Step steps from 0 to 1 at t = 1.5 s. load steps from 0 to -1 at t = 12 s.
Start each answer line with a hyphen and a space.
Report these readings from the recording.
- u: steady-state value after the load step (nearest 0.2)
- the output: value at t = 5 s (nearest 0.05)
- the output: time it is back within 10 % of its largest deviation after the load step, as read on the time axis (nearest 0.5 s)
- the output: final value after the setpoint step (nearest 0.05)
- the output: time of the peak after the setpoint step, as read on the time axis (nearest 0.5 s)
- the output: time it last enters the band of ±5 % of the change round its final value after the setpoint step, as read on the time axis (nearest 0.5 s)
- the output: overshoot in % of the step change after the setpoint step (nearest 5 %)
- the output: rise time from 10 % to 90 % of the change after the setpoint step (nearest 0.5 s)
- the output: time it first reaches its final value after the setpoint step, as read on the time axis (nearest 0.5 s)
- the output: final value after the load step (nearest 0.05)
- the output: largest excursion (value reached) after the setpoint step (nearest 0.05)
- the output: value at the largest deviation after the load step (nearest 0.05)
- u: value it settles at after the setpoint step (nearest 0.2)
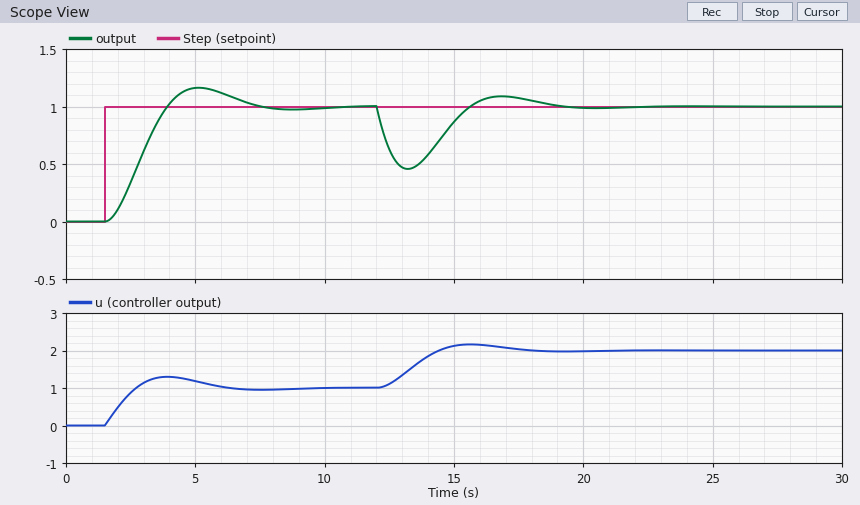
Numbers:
- 2.0
- 1.15
- 18.0 s
- 1.00
- 5.0 s
- 7.0 s
- 15 %
- 1.5 s
- 4.0 s
- 1.00
- 1.15
- 0.45
- 1.0
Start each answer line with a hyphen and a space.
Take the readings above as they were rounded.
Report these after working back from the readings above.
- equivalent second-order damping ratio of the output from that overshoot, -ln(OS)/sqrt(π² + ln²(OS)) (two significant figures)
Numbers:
- 0.52
